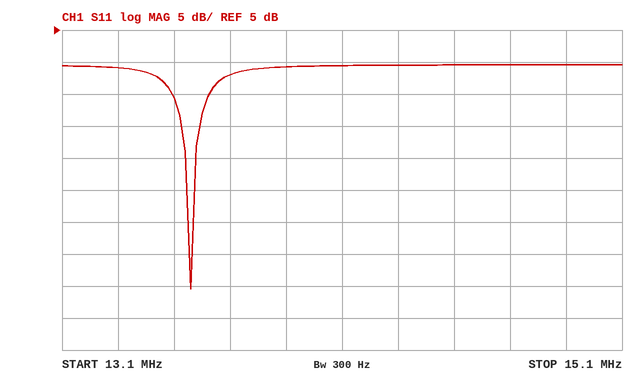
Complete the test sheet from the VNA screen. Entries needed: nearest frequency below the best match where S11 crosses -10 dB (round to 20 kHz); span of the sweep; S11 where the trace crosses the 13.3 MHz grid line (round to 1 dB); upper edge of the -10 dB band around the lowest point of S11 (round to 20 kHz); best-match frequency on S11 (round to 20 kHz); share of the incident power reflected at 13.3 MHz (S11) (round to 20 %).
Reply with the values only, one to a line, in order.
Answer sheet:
13.52 MHz
2 MHz
-1 dB
13.60 MHz
13.56 MHz
80 %
